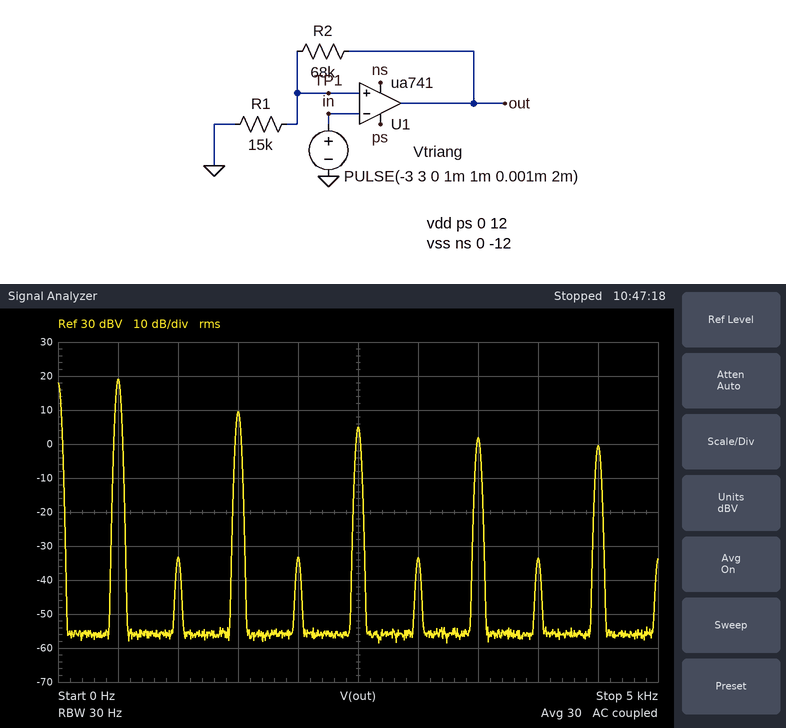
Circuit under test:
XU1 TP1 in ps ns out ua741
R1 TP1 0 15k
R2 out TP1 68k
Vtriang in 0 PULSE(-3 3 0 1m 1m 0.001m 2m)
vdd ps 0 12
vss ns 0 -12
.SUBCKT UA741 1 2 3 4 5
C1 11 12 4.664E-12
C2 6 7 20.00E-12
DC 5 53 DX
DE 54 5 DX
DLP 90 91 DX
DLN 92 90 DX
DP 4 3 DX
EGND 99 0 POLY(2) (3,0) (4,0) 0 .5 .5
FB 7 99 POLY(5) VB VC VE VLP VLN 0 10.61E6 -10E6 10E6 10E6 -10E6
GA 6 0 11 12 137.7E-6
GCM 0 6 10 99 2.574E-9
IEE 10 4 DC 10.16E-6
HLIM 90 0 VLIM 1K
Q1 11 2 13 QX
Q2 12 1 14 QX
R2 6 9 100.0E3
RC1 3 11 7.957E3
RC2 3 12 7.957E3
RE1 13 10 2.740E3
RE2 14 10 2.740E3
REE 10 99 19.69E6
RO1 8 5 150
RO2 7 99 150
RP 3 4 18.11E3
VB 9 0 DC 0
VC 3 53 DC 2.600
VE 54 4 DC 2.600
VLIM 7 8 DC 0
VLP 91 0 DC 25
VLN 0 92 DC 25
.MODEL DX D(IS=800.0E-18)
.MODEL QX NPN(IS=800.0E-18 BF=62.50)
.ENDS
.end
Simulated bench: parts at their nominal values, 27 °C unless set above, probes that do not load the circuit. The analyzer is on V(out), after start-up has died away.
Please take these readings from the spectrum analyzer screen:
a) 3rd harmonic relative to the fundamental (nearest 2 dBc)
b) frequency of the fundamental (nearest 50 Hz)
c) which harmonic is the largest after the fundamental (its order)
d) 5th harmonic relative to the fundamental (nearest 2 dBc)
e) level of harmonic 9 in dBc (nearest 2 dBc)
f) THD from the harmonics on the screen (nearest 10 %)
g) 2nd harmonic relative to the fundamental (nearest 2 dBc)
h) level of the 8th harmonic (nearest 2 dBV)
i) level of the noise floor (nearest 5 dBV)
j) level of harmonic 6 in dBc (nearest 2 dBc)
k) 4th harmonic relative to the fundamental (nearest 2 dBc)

-10 dBc
500 Hz
3
-14 dBc
-20 dBc
40 %
-52 dBc
-34 dBV
-55 dBV
-52 dBc
-52 dBc
